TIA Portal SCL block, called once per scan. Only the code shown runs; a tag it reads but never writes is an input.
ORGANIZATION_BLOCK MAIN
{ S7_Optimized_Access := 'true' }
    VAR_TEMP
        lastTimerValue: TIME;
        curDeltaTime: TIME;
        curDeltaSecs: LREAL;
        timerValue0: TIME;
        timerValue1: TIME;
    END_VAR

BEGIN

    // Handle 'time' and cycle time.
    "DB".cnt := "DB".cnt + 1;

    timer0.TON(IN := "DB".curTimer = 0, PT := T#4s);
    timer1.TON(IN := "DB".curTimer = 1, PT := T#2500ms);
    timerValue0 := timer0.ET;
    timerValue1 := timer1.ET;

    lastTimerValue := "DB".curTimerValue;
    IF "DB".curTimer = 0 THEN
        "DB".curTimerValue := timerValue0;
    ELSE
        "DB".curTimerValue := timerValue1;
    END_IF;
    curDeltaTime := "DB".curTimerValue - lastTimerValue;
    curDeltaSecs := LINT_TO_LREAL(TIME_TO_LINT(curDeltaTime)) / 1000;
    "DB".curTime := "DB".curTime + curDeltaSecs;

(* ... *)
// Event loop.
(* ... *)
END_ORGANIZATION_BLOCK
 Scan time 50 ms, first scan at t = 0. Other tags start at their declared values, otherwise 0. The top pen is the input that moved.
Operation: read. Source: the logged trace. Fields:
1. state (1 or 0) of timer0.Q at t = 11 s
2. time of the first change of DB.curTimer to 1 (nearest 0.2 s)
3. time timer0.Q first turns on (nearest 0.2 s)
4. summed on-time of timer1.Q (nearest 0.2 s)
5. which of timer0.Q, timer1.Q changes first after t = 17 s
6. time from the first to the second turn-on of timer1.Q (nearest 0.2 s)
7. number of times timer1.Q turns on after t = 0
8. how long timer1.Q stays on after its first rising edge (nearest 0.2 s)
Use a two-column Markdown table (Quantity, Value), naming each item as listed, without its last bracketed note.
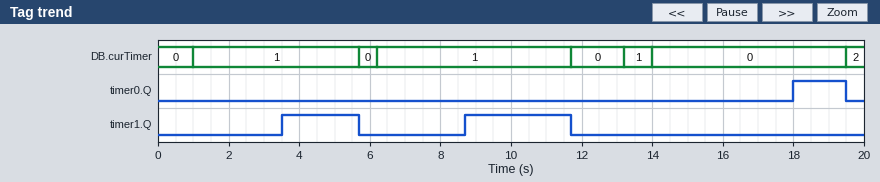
| Quantity | Value |
|---|---|
| state (1 or 0) of timer0.Q at t = 11 s | 0 |
| time of the first change of DB.curTimer to 1 | 1.0 s |
| time timer0.Q first turns on | 18.0 s |
| summed on-time of timer1.Q | 5.2 s |
| which of timer0.Q, timer1.Q changes first after t = 17 s | timer0.Q |
| time from the first to the second turn-on of timer1.Q | 5.2 s |
| number of times timer1.Q turns on after t = 0 | 2 |
| how long timer1.Q stays on after its first rising edge | 2.2 s |
